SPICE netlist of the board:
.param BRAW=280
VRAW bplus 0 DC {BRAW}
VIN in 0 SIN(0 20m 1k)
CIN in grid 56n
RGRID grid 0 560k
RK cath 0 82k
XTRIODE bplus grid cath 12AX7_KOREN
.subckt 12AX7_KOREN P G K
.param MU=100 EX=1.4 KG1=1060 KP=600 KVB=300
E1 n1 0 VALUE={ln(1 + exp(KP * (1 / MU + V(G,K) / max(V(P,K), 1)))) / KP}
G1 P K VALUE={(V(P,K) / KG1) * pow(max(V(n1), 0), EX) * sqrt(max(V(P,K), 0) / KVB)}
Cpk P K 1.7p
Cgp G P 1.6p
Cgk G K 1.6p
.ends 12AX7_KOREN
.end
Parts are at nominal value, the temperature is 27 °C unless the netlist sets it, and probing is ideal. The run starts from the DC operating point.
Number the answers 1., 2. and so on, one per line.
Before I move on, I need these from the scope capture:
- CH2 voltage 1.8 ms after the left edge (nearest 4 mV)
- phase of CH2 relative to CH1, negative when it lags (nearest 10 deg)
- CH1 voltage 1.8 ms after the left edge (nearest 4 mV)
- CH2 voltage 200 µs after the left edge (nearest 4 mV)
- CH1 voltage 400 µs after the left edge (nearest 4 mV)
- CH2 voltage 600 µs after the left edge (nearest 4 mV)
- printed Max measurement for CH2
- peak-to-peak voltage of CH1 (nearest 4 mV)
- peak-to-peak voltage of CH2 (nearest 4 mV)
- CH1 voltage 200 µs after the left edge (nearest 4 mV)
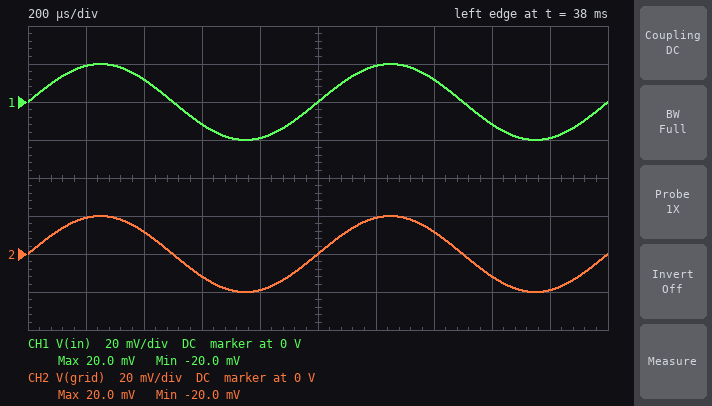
1. -20 mV
2. 0 deg
3. -20 mV
4. 20 mV
5. 12 mV
6. -12 mV
7. 20.0 mV
8. 40 mV
9. 40 mV
10. 20 mV
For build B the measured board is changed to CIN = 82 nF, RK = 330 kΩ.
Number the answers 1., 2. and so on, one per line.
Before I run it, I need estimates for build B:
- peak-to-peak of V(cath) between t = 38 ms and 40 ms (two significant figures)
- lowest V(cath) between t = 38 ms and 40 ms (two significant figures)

1. 35 mV
2. 3.1 V
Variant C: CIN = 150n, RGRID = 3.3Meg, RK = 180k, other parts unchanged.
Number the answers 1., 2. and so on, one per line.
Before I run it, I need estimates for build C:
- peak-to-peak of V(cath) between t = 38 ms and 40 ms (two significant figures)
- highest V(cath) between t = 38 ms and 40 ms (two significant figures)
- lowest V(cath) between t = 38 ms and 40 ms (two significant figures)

1. 34 mV
2. 2.9 V
3. 2.8 V
